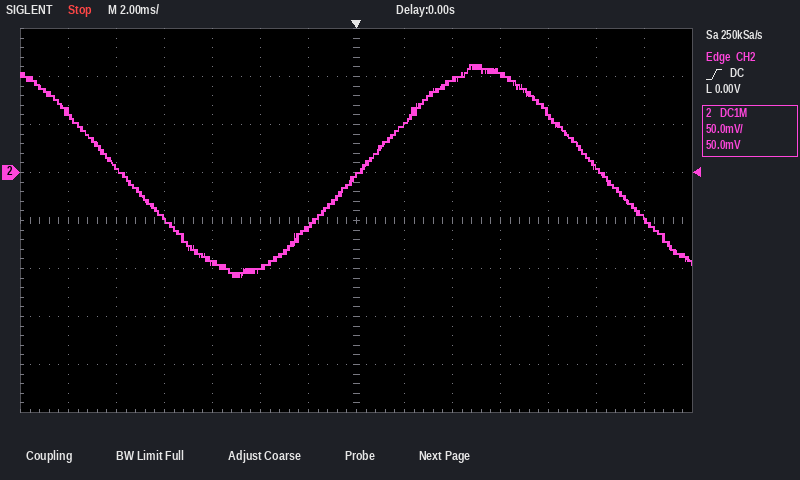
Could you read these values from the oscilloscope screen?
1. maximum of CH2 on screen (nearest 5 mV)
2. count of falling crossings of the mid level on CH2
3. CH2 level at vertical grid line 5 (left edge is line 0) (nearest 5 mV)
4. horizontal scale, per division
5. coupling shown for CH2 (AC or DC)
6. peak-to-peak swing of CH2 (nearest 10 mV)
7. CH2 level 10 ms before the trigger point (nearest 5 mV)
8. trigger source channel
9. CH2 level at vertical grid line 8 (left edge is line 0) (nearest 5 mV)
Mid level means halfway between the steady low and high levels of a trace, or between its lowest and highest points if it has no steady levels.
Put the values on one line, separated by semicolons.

110 mV; 2; -100 mV; 2 ms; DC; 220 mV; 5 mV; CH2; 50 mV
